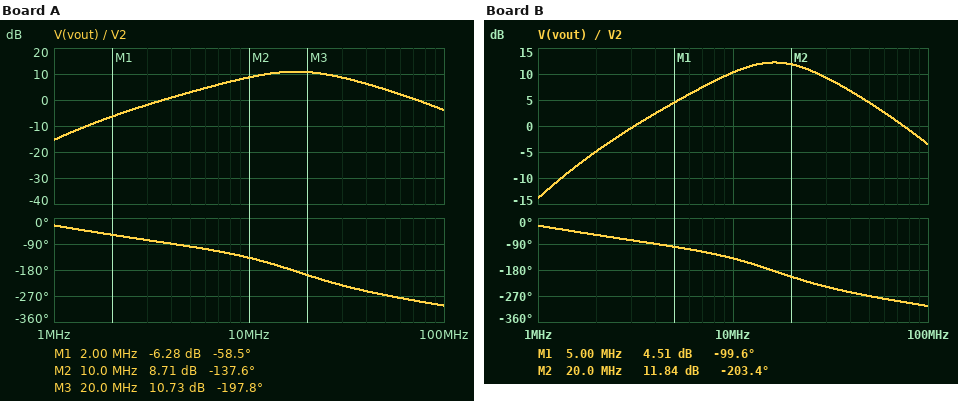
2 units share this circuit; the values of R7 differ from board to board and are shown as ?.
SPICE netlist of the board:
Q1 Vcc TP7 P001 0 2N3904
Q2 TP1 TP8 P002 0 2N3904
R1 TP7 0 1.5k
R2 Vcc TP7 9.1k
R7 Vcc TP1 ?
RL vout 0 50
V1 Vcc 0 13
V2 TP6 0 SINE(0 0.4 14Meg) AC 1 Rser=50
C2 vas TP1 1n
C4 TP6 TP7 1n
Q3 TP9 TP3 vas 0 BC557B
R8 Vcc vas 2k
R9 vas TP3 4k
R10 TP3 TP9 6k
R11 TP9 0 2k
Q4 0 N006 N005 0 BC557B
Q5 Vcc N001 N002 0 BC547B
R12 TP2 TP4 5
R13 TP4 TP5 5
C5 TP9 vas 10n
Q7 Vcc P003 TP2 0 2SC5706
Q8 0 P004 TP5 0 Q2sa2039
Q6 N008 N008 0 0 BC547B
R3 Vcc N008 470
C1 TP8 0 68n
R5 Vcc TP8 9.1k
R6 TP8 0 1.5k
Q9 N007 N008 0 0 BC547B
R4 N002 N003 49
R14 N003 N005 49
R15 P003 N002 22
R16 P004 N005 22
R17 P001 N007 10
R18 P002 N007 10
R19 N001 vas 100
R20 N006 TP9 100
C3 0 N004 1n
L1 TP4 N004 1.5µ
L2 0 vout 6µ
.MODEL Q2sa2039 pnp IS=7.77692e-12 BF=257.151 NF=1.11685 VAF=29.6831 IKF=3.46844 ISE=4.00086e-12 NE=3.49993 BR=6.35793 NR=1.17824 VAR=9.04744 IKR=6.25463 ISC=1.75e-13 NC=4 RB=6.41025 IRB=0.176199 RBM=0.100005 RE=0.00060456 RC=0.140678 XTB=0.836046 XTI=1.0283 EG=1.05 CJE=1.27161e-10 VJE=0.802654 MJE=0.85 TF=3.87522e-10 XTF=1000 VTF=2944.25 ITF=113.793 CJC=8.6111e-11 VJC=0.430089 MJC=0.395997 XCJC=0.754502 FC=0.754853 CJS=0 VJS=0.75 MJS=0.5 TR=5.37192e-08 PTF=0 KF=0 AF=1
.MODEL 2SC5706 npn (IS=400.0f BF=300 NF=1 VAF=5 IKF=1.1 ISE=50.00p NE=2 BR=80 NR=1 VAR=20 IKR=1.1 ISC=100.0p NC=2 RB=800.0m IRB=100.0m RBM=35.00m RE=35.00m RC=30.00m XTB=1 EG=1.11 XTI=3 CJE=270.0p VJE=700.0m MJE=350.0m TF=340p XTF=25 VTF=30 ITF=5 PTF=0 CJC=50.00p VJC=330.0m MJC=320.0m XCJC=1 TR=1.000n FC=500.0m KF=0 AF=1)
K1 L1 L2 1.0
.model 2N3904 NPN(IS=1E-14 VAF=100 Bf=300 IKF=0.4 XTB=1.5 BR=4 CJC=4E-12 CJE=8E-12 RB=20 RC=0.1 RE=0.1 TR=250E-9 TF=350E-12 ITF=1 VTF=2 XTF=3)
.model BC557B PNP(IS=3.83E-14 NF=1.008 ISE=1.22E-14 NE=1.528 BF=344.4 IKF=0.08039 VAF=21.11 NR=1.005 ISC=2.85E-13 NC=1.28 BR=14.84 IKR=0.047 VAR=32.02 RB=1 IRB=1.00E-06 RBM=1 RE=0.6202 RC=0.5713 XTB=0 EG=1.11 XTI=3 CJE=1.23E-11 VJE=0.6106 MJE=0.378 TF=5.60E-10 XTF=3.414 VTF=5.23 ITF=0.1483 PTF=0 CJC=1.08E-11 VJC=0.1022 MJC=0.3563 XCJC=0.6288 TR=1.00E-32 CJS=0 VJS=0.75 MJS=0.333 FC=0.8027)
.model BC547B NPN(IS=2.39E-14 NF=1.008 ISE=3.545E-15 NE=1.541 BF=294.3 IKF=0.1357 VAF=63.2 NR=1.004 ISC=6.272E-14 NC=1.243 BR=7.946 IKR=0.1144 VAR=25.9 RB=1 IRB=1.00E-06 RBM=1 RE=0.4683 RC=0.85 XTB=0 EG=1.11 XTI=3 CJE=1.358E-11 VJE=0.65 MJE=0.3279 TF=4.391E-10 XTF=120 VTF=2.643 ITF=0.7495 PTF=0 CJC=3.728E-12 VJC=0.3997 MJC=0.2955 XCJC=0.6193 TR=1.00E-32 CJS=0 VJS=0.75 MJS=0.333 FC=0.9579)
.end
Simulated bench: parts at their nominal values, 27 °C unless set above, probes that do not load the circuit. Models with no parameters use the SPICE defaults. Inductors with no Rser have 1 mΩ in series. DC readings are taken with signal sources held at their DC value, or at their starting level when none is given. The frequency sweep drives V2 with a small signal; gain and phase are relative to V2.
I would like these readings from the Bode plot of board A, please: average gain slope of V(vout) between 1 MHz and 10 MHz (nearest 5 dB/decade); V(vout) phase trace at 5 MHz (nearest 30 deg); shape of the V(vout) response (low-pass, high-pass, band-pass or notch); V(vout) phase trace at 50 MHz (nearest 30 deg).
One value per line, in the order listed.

25 dB/decade
-90 deg
band-pass
-270 deg
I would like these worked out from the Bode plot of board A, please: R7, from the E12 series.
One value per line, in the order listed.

180 Ω
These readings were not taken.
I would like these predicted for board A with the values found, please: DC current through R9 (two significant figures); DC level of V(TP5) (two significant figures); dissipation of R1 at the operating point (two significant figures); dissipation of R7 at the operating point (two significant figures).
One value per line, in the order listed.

160 µA
6.5 V
2.1 mW
30 mW
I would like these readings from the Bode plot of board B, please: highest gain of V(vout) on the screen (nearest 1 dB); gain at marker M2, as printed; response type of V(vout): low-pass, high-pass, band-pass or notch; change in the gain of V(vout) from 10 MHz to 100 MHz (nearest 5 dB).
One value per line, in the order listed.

12 dB
11.84 dB
band-pass
-15 dB
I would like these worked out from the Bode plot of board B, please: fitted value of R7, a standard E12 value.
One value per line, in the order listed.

220 Ω
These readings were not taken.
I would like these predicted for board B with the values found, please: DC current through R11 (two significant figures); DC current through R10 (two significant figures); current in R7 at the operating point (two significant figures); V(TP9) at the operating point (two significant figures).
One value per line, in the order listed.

2.8 mA
170 µA
13 mA
5.7 V
